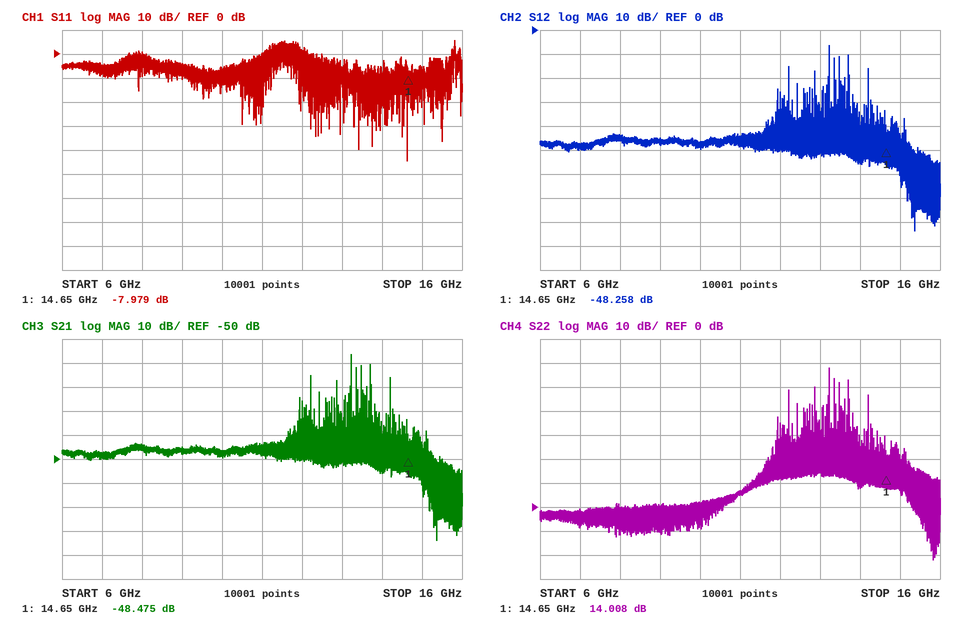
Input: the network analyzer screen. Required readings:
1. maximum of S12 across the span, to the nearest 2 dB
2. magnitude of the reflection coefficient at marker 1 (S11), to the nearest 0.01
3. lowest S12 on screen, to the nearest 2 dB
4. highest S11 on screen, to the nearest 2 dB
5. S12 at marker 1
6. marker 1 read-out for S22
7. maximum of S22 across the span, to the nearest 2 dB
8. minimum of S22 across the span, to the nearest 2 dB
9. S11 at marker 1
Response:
-6 dB
0.40
-84 dB
6 dB
-48.258 dB
14.008 dB
58 dB
-22 dB
-7.979 dB
